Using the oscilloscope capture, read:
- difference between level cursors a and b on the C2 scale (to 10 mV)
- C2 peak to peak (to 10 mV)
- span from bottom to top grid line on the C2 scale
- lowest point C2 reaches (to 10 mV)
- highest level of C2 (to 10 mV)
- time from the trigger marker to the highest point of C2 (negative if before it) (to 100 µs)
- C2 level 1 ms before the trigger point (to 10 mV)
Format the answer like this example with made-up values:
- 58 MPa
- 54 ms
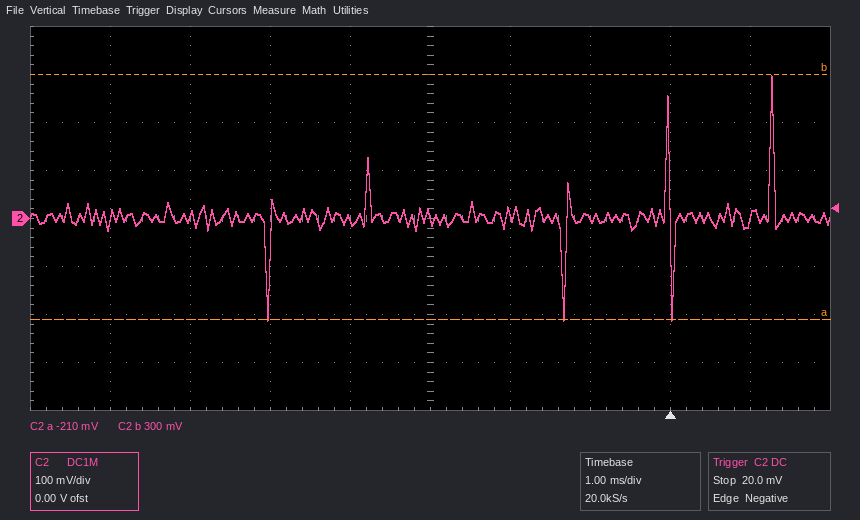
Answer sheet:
- 510 mV
- 510 mV
- 800 mV
- -210 mV
- 300 mV
- +1.3 ms
- 0 mV
